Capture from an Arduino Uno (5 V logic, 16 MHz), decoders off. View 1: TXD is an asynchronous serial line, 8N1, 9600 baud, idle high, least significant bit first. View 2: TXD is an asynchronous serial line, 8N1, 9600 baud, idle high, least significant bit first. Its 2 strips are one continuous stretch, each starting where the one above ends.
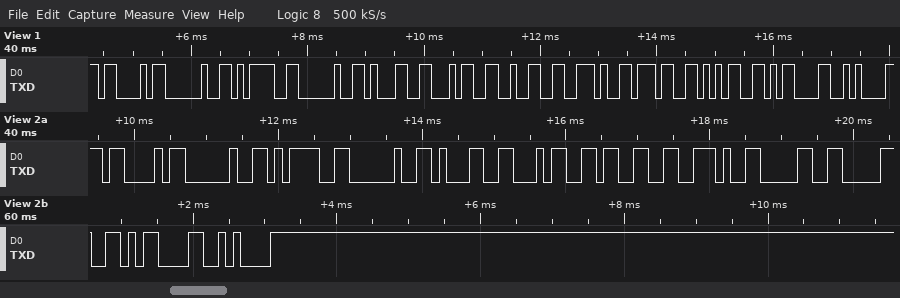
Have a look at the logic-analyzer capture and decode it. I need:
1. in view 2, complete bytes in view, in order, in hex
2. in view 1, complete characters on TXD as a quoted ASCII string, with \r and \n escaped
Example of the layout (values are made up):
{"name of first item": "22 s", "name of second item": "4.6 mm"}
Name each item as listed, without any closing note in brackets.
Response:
{"in view 2, complete bytes in view, in order, in hex": "43 20 3D 20 31 34 33 2E 30 30 0D 0A", "in view 1, complete characters on TXD as a quoted ASCII string, with \\r and \\n escaped": "\"C = 142.75\\r\\n\""}
